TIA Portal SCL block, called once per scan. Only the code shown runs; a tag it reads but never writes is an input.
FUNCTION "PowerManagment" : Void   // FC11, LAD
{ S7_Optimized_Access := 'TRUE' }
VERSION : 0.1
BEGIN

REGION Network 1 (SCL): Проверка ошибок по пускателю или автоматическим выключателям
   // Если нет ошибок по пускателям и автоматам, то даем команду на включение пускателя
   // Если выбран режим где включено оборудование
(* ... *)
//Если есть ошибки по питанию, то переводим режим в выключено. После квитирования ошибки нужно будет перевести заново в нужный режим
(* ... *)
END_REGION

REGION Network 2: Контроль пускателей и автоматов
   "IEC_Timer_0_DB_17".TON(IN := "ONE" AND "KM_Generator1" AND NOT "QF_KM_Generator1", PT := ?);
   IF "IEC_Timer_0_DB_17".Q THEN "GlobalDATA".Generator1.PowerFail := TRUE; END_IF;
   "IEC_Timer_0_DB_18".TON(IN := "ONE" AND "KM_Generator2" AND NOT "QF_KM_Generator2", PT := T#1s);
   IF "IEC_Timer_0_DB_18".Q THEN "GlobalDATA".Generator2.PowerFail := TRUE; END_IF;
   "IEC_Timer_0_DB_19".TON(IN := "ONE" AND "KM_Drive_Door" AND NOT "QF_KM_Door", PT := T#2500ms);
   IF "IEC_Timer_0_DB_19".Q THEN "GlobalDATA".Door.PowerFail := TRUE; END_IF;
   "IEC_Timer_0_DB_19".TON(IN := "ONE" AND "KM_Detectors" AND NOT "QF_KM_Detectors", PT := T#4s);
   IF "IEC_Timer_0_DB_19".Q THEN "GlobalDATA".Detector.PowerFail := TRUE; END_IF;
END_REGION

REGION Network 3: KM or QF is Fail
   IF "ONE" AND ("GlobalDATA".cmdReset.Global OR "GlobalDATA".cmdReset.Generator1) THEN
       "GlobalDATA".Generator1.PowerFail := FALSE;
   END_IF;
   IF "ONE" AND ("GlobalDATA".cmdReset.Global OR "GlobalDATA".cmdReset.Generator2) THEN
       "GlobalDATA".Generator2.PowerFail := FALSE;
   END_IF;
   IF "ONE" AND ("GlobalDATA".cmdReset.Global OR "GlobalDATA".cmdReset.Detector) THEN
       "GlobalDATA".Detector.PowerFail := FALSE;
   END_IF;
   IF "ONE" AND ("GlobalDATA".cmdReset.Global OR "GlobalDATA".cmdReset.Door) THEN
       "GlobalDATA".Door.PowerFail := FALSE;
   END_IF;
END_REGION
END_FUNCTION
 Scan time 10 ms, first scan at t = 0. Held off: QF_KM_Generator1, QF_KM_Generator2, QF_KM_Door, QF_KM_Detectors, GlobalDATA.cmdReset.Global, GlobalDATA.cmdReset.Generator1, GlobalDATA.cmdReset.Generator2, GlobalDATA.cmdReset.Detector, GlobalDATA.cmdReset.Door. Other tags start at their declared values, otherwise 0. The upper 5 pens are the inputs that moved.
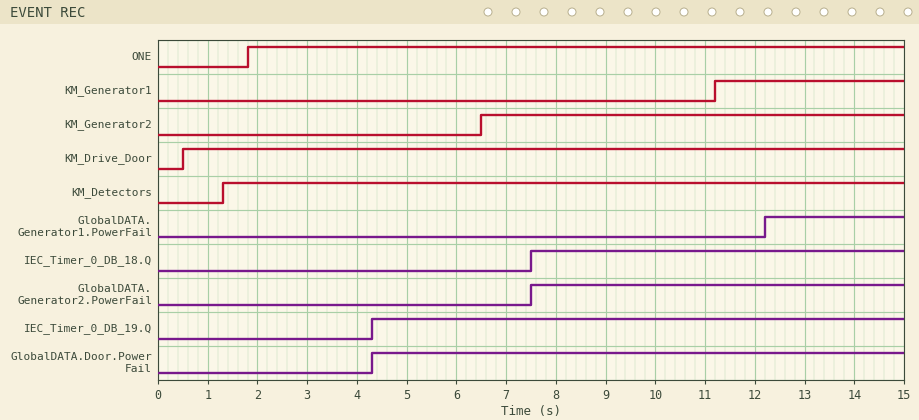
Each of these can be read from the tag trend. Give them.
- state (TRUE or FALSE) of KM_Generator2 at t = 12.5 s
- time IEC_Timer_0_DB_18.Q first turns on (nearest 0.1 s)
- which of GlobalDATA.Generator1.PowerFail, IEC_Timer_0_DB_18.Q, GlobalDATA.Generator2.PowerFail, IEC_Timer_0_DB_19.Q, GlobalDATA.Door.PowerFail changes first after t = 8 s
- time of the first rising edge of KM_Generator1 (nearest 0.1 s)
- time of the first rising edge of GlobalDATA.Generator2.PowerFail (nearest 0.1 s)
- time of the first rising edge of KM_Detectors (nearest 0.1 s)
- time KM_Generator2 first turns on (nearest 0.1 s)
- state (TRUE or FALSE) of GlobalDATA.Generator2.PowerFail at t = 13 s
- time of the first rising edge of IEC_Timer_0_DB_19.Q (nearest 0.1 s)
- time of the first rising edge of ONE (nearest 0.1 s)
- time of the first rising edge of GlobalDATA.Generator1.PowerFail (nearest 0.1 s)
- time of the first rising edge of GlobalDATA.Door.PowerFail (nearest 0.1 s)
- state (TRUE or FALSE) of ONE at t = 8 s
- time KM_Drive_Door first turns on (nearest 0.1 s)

TRUE
7.5 s
GlobalDATA.Generator1.PowerFail
11.2 s
7.5 s
1.3 s
6.5 s
TRUE
4.3 s
1.8 s
12.2 s
4.3 s
TRUE
0.5 s
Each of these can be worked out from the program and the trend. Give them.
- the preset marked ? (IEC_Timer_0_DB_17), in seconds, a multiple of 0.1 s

1.0 s
